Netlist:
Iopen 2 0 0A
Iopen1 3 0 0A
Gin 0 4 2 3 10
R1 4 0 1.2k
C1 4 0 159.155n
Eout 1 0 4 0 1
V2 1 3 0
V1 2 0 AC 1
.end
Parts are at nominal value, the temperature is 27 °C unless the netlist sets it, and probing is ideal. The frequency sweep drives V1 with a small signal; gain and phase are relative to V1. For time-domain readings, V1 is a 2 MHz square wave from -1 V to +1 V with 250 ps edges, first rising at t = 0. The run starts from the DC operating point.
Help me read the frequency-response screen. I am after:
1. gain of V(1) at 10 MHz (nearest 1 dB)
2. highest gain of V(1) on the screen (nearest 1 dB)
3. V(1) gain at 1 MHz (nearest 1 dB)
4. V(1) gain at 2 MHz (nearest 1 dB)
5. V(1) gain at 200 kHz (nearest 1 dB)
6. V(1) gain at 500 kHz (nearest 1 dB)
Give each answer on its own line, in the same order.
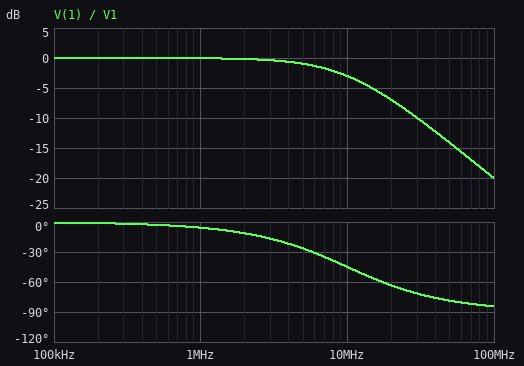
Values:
-3 dB
0 dB
0 dB
0 dB
0 dB
0 dB
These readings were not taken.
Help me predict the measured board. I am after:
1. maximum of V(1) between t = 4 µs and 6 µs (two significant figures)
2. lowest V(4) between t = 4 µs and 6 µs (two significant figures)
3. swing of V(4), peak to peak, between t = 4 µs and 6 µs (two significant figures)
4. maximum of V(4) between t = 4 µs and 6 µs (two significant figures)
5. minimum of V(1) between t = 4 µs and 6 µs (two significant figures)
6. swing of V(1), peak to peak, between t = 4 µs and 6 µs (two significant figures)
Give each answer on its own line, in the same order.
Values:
1.0 V
-1.0 V
2.0 V
1.0 V
-1.0 V
2.0 V
